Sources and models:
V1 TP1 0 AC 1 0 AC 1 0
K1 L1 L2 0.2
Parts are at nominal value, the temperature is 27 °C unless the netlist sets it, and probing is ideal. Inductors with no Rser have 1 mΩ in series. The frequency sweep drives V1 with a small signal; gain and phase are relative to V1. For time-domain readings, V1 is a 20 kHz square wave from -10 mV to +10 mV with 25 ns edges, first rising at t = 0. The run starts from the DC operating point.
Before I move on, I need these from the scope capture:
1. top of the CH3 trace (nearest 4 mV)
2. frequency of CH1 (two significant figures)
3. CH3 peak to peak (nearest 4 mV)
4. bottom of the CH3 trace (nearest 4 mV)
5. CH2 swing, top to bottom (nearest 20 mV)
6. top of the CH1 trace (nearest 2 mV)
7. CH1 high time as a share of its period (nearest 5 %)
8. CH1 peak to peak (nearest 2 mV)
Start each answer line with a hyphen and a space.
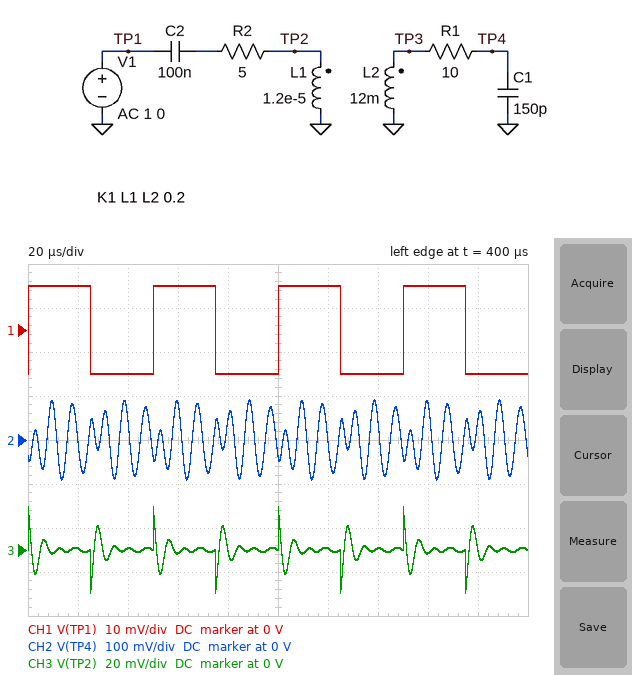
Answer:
- 20 mV
- 20 kHz
- 40 mV
- -20 mV
- 180 mV
- 10 mV
- 50 %
- 20 mV
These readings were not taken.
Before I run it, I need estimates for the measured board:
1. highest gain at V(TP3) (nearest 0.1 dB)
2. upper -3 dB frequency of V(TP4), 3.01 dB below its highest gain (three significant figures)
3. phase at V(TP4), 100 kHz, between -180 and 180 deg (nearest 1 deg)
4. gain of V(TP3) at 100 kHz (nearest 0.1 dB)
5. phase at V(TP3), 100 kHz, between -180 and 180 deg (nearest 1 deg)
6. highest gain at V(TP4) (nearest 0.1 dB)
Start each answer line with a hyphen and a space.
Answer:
- 46.9 dB
- 119 kHz
- 147 deg
- 25.1 dB
- 147 deg
- 46.9 dB
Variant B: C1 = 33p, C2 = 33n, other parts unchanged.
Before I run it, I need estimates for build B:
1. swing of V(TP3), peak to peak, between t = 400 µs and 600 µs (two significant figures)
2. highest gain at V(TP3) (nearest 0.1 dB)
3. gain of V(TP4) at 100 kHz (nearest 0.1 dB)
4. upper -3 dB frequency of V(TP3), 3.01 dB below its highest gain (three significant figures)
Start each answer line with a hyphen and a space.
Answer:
- 550 mV
- 44.6 dB
- 2.8 dB
- 279 kHz
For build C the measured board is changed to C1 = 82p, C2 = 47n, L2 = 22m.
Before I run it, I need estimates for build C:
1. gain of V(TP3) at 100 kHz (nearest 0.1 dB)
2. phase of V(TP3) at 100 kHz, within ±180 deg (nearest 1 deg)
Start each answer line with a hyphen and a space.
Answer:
- 18.7 dB
- 169 deg
